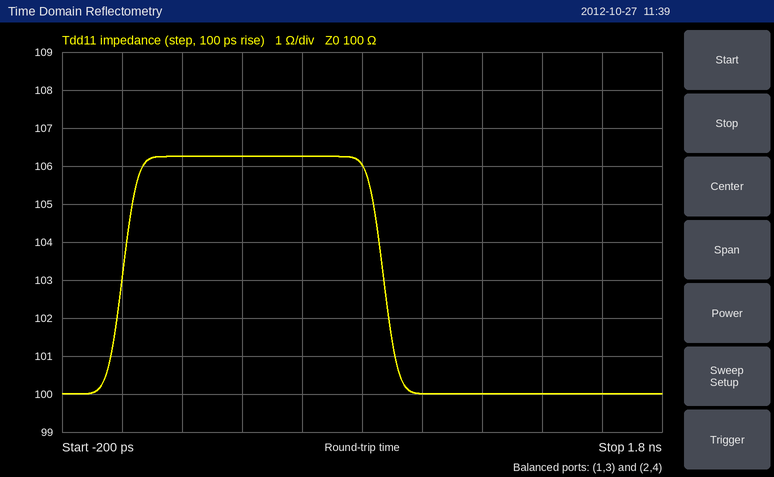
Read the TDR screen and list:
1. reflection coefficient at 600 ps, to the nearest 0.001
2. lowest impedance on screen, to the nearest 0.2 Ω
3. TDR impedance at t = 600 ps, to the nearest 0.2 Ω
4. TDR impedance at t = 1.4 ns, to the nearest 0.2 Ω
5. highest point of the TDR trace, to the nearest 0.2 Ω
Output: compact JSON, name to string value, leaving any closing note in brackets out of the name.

{"reflection coefficient at 600 ps, to the nearest 0.001": "+0.030", "lowest impedance on screen, to the nearest 0.2 Ω": "100.0 Ω", "TDR impedance at t = 600 ps, to the nearest 0.2 Ω": "106.2 Ω", "TDR impedance at t = 1.4 ns, to the nearest 0.2 Ω": "100.0 Ω", "highest point of the TDR trace, to the nearest 0.2 Ω": "106.2 Ω"}
